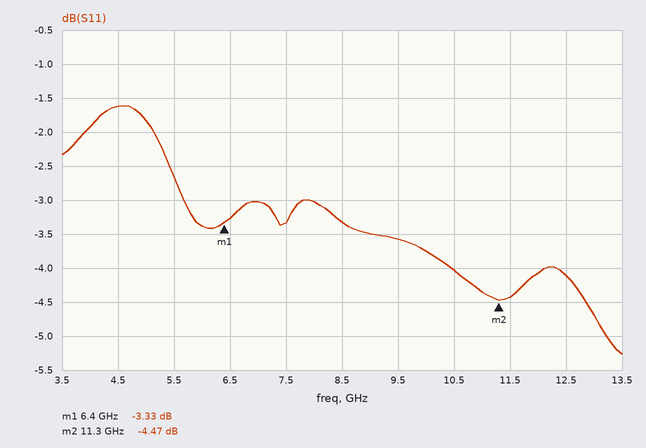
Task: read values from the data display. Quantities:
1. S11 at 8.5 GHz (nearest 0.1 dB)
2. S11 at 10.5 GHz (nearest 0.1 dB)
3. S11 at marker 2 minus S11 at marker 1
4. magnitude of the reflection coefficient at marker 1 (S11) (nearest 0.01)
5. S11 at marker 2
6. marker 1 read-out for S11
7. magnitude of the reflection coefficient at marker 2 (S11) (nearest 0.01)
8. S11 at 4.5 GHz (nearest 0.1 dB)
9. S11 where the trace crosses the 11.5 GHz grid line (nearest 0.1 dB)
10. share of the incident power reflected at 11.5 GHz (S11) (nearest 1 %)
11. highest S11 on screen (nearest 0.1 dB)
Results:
-3.3 dB
-4.0 dB
-1.14 dB
0.68
-4.47 dB
-3.33 dB
0.60
-1.6 dB
-4.4 dB
36 %
-1.6 dB
